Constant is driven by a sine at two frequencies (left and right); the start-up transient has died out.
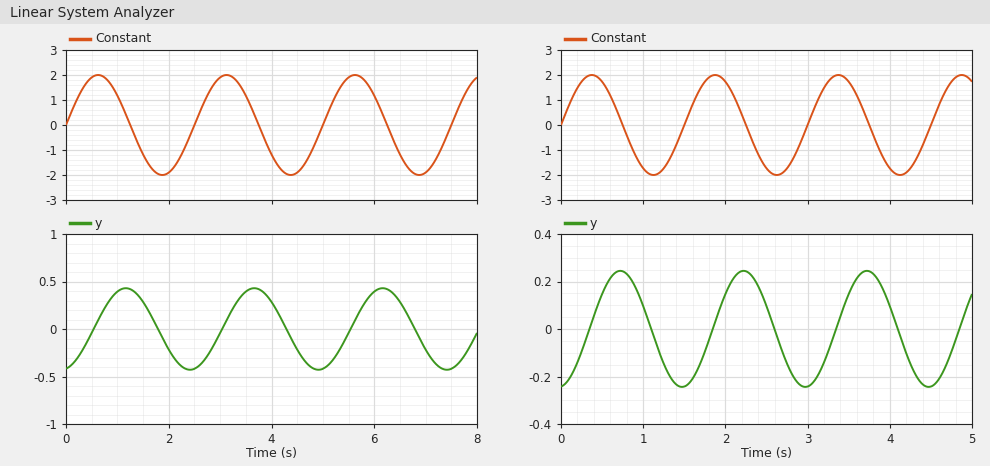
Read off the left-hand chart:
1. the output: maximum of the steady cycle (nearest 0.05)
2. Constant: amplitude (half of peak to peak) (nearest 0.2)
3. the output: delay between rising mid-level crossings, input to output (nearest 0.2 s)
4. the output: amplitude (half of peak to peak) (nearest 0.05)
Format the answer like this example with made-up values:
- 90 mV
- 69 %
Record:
- 0.45
- 2.0
- 0.6 s
- 0.45
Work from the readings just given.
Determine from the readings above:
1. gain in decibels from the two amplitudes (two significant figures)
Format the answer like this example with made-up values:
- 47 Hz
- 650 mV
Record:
- -13 dB
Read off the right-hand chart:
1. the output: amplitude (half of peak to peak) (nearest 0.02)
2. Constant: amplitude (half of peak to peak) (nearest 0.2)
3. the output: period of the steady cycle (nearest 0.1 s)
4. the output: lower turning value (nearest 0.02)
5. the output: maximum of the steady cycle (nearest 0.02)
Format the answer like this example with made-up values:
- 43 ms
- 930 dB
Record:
- 0.24
- 2.0
- 1.5 s
- -0.24
- 0.24
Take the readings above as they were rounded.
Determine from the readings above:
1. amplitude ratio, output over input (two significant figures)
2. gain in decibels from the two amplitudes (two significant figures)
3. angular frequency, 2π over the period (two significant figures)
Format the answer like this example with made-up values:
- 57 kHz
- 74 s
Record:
- 0.12
- -18 dB
- 4.2 rad/s
